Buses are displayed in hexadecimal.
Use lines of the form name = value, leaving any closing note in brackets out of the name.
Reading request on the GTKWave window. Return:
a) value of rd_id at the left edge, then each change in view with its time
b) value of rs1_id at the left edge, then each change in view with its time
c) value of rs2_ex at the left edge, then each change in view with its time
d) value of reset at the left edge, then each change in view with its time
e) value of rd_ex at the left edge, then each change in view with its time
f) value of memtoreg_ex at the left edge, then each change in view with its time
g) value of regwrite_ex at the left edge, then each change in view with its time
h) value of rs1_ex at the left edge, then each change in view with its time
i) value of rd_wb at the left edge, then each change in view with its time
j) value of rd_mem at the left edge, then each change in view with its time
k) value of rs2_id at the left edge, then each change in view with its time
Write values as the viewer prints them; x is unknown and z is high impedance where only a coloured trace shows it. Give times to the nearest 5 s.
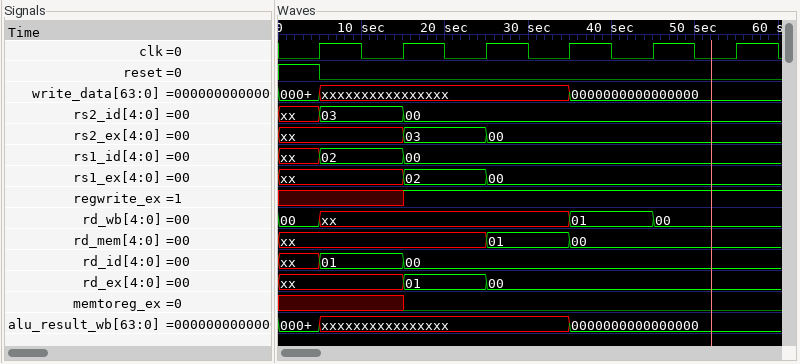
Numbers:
value of rd_id at the left edge, then each change in view with its time = xx, 01 at 5 s, 00 at 15 s
value of rs1_id at the left edge, then each change in view with its time = xx, 02 at 5 s, 00 at 15 s
value of rs2_ex at the left edge, then each change in view with its time = xx, 03 at 15 s, 00 at 25 s
value of reset at the left edge, then each change in view with its time = 1, 0 at 5 s
value of rd_ex at the left edge, then each change in view with its time = xx, 01 at 15 s, 00 at 25 s
value of memtoreg_ex at the left edge, then each change in view with its time = x, 0 at 15 s
value of regwrite_ex at the left edge, then each change in view with its time = x, 1 at 15 s
value of rs1_ex at the left edge, then each change in view with its time = xx, 02 at 15 s, 00 at 25 s
value of rd_wb at the left edge, then each change in view with its time = 00, xx at 5 s, 01 at 35 s, 00 at 45 s
value of rd_mem at the left edge, then each change in view with its time = xx, 01 at 25 s, 00 at 35 s
value of rs2_id at the left edge, then each change in view with its time = xx, 03 at 5 s, 00 at 15 s
